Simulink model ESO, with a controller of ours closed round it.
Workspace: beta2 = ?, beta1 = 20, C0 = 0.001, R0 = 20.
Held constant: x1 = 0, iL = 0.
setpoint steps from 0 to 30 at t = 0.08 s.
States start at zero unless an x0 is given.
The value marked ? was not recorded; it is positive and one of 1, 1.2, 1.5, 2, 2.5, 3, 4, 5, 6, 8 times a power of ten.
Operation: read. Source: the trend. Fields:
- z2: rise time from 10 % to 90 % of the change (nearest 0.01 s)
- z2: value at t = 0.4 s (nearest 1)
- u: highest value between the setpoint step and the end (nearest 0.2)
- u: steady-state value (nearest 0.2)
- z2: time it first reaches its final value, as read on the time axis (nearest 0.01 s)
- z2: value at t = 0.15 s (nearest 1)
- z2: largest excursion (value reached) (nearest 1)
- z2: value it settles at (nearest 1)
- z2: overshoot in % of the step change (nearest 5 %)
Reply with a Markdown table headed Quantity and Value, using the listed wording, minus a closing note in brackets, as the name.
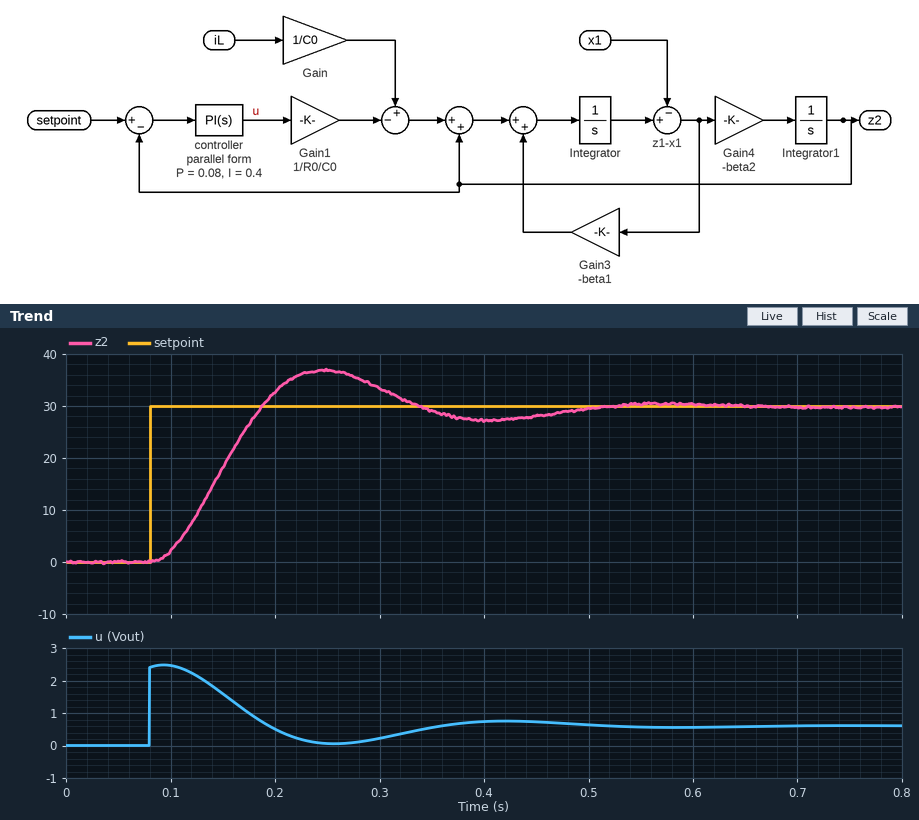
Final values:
| Quantity | Value |
|---|---|
| z2: rise time from 10 % to 90 % of the change | 0.07 s |
| z2: value at t = 0.4 s | 27 |
| u: highest value between the setpoint step and the end | 2.4 |
| u: steady-state value | 0.6 |
| z2: time it first reaches its final value, as read on the time axis | 0.19 s |
| z2: value at t = 0.15 s | 18 |
| z2: largest excursion (value reached) | 37 |
| z2: value it settles at | 30 |
| z2: overshoot in % of the step change | 25 % |
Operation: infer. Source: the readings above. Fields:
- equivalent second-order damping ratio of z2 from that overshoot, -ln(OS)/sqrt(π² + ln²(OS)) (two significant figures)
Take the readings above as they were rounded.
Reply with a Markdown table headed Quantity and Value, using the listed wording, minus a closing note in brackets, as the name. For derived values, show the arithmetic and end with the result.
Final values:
| Quantity | Value |
|---|---|
| equivalent second-order damping ratio of z2 from that overshoot, -ln(OS)/sqrt(π² + ln²(OS)) | ln(0.25) = -1.386; 1.386 / sqrt(9.870 + 1.922) = 0.40 |
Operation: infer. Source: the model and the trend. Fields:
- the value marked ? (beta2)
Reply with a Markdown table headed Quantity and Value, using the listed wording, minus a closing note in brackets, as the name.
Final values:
| Quantity | Value |
|---|---|
| the value marked ? | 100 |
